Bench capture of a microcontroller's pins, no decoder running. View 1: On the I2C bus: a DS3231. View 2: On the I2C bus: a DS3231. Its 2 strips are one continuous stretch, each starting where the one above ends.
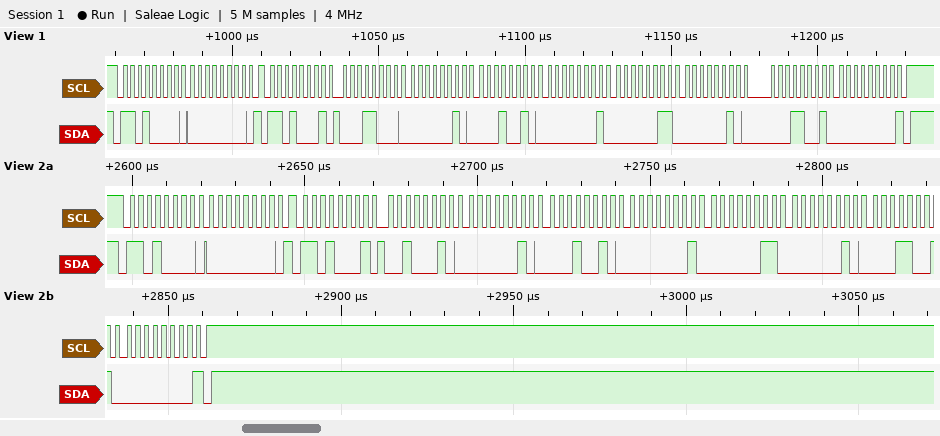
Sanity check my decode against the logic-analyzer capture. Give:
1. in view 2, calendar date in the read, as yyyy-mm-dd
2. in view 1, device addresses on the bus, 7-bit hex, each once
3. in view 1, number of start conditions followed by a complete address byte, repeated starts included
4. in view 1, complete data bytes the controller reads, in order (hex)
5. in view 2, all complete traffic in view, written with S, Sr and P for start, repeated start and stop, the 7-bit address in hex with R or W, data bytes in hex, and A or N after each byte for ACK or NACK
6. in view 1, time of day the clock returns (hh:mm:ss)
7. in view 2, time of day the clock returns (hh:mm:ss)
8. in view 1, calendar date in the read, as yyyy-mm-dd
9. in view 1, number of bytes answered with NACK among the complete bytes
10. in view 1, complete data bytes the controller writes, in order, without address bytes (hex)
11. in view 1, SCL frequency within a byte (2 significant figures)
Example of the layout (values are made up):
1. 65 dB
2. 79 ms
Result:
1. 2019-02-03
2. 0x68
3. 2
4. 18 02 12 01 03 02 19 00
5. S 68W A 00 A Sr 68R A 22 A 02 A 12 A 01 A 03 A 02 A 19 A 00 N P
6. 12:02:18
7. 12:02:22
8. 2019-02-03
9. 1
10. 00
11. 400 kHz
